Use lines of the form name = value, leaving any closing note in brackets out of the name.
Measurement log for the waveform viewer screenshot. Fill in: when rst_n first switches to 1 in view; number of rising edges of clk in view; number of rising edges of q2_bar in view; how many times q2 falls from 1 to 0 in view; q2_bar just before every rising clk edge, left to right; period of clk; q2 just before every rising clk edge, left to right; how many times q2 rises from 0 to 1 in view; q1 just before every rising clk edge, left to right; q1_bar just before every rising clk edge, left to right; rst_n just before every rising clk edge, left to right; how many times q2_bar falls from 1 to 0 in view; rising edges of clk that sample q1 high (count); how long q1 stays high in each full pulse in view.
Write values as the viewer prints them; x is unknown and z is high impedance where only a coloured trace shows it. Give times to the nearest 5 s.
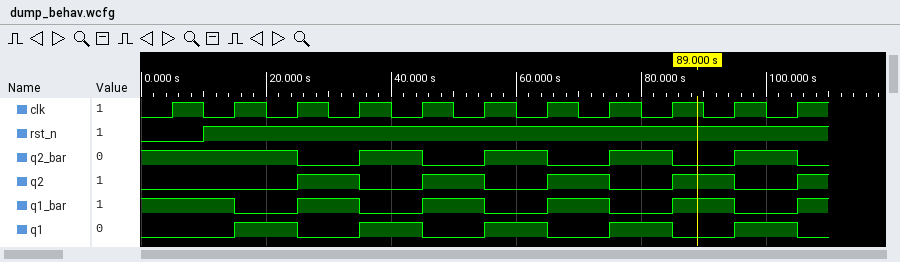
when rst_n first switches to 1 in view = 10 s
number of rising edges of clk in view = 11
number of rising edges of q2_bar in view = 4
how many times q2 falls from 1 to 0 in view = 4
q2_bar just before every rising clk edge, left to right = 1 1 1 0 1 0 1 0 1 0 1
period of clk = 10 s
q2 just before every rising clk edge, left to right = 0 0 0 1 0 1 0 1 0 1 0
how many times q2 rises from 0 to 1 in view = 5
q1 just before every rising clk edge, left to right = 0 0 1 0 1 0 1 0 1 0 1
q1_bar just before every rising clk edge, left to right = 1 1 0 1 0 1 0 1 0 1 0
rst_n just before every rising clk edge, left to right = 0 1 1 1 1 1 1 1 1 1 1
how many times q2_bar falls from 1 to 0 in view = 5
rising edges of clk that sample q1 high = 5
how long q1 stays high in each full pulse in view = 10 s, 10 s, 10 s, 10 s, 10 s
